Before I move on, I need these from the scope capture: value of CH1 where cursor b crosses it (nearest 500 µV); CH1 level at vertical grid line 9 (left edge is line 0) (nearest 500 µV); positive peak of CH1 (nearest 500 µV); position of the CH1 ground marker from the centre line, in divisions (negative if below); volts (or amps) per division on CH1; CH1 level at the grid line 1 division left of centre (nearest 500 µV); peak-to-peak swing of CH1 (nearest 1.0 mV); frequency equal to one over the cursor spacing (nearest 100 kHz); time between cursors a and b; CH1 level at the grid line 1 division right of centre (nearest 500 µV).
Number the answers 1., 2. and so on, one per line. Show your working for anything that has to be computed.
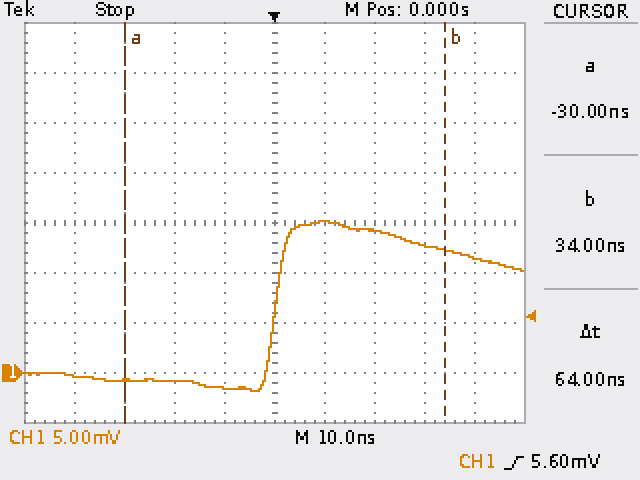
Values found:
1. 12.5 mV
2. 11.5 mV
3. 15.0 mV
4. -3.0 div
5. 5 mV
6. -1.5 mV
7. 17.0 mV
8. 1 / 64 ns ≈ 15.6 MHz
9. 64 ns
10. 15.0 mV
